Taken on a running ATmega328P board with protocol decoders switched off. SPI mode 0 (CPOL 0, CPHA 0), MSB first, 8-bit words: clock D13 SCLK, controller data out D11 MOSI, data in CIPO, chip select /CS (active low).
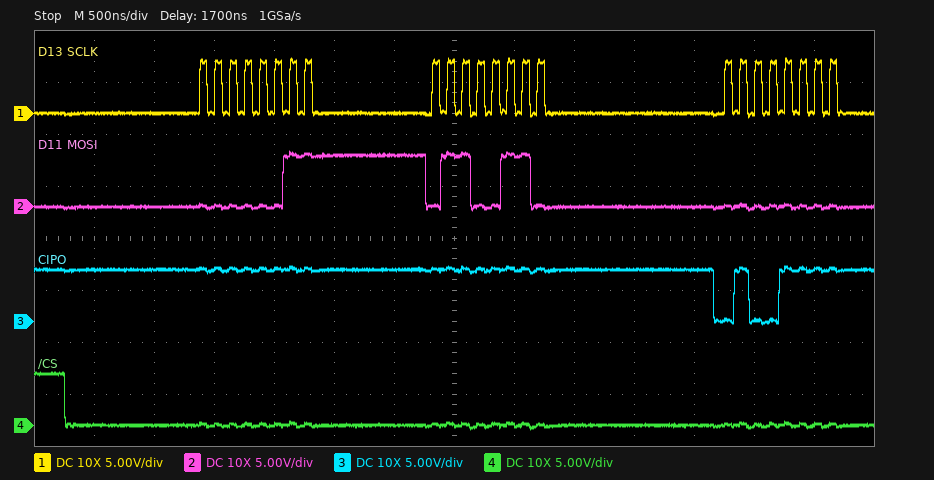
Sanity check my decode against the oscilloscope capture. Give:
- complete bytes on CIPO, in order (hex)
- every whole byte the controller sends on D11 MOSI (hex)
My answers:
FF FF 4F
03 66 00
